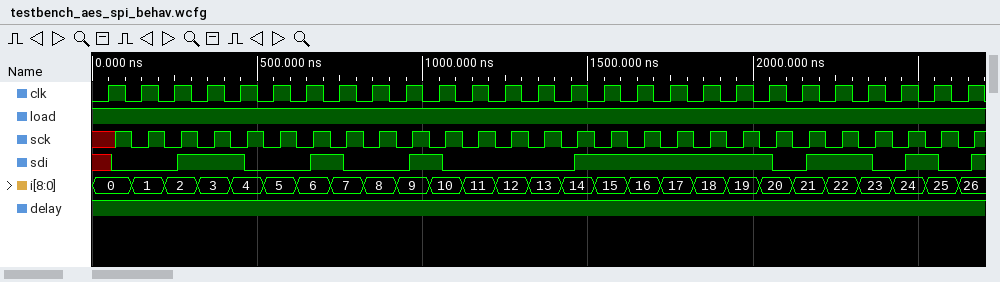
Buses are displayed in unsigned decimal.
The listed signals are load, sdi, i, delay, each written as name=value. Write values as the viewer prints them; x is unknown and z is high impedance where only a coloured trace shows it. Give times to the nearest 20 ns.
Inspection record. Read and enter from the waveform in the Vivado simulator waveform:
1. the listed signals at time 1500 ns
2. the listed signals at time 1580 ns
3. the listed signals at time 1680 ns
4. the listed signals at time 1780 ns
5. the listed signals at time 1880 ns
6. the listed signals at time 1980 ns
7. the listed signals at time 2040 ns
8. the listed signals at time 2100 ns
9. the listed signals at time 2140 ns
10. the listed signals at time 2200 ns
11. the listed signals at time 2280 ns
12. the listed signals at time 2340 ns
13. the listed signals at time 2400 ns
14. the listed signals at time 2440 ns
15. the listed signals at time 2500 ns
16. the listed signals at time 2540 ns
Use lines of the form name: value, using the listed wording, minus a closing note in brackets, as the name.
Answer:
the listed signals at time 1500 ns: load=1, sdi=1, i=14, delay=1
the listed signals at time 1580 ns: load=1, sdi=1, i=15, delay=1
the listed signals at time 1680 ns: load=1, sdi=1, i=16, delay=1
the listed signals at time 1780 ns: load=1, sdi=1, i=17, delay=1
the listed signals at time 1880 ns: load=1, sdi=1, i=18, delay=1
the listed signals at time 1980 ns: load=1, sdi=1, i=19, delay=1
the listed signals at time 2040 ns: load=1, sdi=1, i=20, delay=1
the listed signals at time 2100 ns: load=1, sdi=0, i=20, delay=1
the listed signals at time 2140 ns: load=1, sdi=0, i=21, delay=1
the listed signals at time 2200 ns: load=1, sdi=1, i=21, delay=1
the listed signals at time 2280 ns: load=1, sdi=1, i=22, delay=1
the listed signals at time 2340 ns: load=1, sdi=1, i=23, delay=1
the listed signals at time 2400 ns: load=1, sdi=0, i=23, delay=1
the listed signals at time 2440 ns: load=1, sdi=0, i=24, delay=1
the listed signals at time 2500 ns: load=1, sdi=1, i=24, delay=1
the listed signals at time 2540 ns: load=1, sdi=1, i=25, delay=1
